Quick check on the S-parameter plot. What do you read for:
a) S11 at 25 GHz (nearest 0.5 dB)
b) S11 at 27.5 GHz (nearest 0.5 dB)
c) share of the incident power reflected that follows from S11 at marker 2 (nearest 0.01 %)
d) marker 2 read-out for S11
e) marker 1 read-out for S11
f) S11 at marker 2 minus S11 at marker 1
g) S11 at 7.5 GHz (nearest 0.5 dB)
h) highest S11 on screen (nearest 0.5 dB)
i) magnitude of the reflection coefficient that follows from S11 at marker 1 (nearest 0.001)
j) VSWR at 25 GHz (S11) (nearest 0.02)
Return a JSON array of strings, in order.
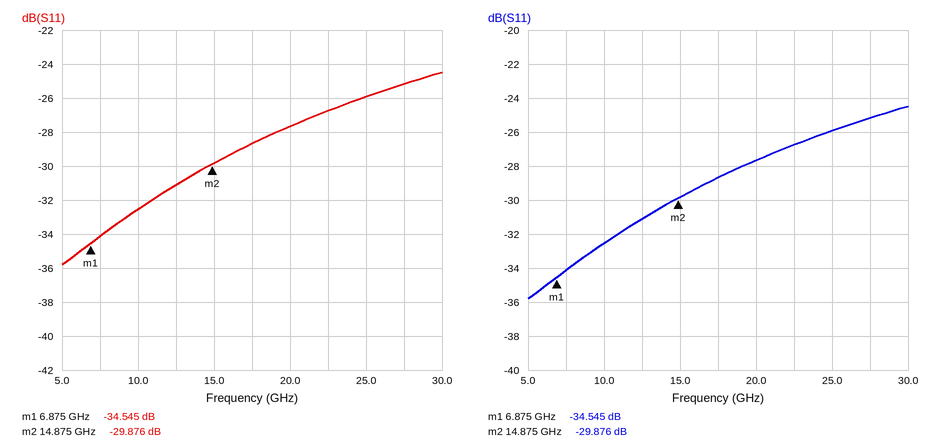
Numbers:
["-26.0 dB", "-25.0 dB", "0.10 %", "-29.876 dB", "-34.545 dB", "4.669 dB", "-34.0 dB", "-24.5 dB", "0.019", "1.10"]
